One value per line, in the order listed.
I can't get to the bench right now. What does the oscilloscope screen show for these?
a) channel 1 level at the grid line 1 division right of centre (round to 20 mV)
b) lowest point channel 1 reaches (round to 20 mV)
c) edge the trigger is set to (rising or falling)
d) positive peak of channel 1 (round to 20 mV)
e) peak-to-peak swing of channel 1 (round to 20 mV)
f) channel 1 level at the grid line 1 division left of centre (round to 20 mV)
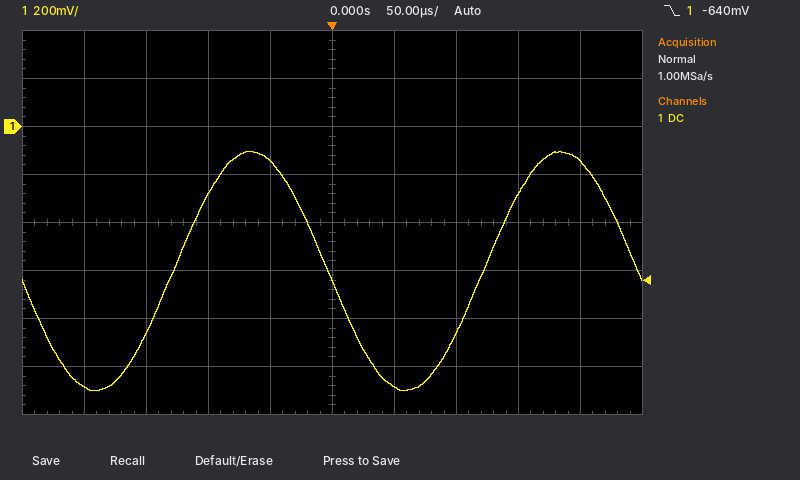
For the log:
-1.08 V
-1.10 V
falling
-100 mV
1.00 V
-140 mV
